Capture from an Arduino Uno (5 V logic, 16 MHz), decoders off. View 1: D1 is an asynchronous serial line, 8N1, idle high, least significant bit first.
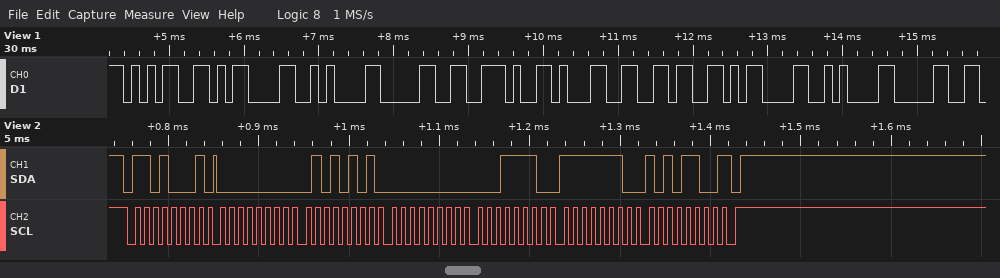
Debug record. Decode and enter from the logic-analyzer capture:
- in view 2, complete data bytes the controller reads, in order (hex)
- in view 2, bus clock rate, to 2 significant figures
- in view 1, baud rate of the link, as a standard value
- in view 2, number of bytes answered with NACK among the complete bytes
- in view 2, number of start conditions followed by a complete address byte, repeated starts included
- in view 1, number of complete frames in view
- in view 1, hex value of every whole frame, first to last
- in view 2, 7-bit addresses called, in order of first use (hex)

00 55 00 1E FE AC
100 kHz
9600 baud
1
1
10
35 0D 0A 30 2E 31 36 0D 0A 30
0x68
